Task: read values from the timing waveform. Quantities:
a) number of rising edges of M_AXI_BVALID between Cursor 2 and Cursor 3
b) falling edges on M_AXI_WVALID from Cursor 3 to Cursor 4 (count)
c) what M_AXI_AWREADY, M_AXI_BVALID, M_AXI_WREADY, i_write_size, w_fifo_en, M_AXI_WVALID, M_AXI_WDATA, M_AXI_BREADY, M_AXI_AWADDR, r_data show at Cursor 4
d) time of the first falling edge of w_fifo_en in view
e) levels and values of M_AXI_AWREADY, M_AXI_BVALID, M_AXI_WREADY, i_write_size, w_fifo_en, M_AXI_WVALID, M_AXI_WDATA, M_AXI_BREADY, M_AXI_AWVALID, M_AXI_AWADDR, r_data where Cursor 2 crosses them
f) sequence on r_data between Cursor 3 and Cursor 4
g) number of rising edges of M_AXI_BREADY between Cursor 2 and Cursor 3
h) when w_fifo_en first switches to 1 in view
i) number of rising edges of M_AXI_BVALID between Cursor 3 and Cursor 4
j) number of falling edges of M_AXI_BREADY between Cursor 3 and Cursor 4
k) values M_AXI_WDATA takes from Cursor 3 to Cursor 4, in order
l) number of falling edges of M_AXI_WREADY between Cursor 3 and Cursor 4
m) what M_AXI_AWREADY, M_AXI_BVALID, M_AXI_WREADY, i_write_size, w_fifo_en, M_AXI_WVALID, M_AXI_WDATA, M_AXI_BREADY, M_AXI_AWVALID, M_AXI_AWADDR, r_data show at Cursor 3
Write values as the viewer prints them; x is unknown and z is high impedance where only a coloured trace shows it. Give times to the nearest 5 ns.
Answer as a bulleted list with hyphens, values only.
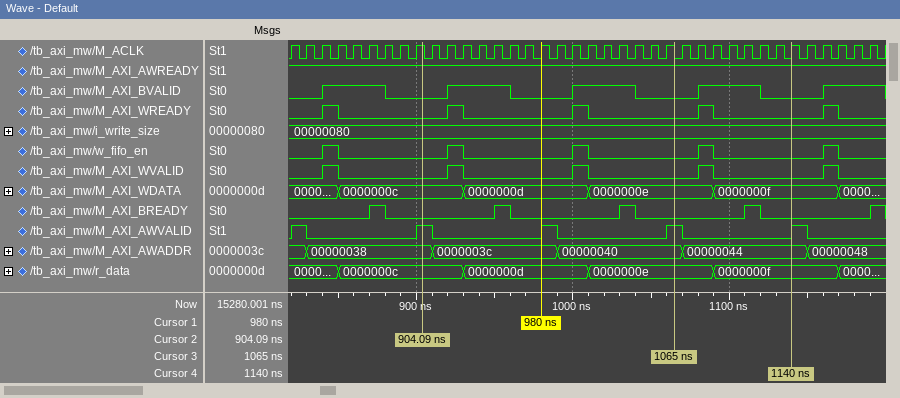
- 2
- 1
- M_AXI_AWREADY=1, M_AXI_BVALID=0, M_AXI_WREADY=0, i_write_size=00000080, w_fifo_en=0, M_AXI_WVALID=0, M_AXI_WDATA=0000000f, M_AXI_BREADY=0, M_AXI_AWADDR=00000044, r_data=0000000f
- 850 ns
- M_AXI_AWREADY=1, M_AXI_BVALID=0, M_AXI_WREADY=0, i_write_size=00000080, w_fifo_en=0, M_AXI_WVALID=0, M_AXI_WDATA=0000000c, M_AXI_BREADY=0, M_AXI_AWVALID=1, M_AXI_AWADDR=00000038, r_data=0000000c
- 0000000e, 0000000f
- 2
- 840 ns
- 1
- 1
- 0000000e, 0000000f
- 1
- M_AXI_AWREADY=1, M_AXI_BVALID=0, M_AXI_WREADY=0, i_write_size=00000080, w_fifo_en=0, M_AXI_WVALID=0, M_AXI_WDATA=0000000e, M_AXI_BREADY=0, M_AXI_AWVALID=1, M_AXI_AWADDR=00000040, r_data=0000000e
